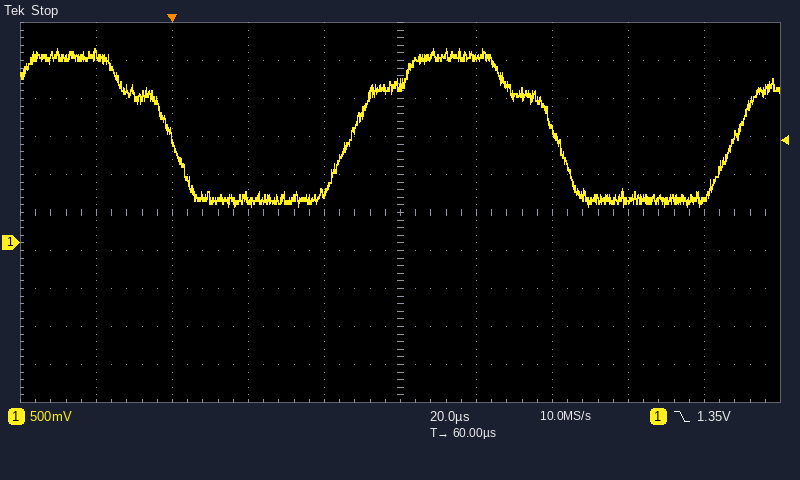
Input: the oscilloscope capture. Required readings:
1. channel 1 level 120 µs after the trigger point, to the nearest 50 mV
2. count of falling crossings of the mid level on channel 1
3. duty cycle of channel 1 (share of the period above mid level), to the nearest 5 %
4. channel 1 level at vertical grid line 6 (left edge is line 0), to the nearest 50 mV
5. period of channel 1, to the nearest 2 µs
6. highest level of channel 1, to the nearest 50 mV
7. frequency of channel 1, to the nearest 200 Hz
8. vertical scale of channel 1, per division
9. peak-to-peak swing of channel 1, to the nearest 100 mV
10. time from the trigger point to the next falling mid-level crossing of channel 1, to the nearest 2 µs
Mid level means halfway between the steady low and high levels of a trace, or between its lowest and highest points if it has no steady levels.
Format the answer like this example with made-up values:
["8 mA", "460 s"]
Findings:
["550 mV", "2", "50 %", "2.45 V", "102 µs", "2.55 V", "9.8 kHz", "500 mV", "2.10 V", "100 µs"]
